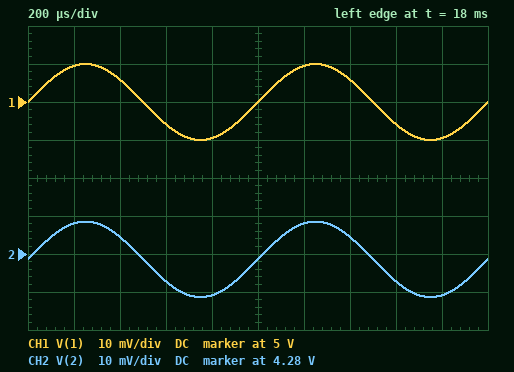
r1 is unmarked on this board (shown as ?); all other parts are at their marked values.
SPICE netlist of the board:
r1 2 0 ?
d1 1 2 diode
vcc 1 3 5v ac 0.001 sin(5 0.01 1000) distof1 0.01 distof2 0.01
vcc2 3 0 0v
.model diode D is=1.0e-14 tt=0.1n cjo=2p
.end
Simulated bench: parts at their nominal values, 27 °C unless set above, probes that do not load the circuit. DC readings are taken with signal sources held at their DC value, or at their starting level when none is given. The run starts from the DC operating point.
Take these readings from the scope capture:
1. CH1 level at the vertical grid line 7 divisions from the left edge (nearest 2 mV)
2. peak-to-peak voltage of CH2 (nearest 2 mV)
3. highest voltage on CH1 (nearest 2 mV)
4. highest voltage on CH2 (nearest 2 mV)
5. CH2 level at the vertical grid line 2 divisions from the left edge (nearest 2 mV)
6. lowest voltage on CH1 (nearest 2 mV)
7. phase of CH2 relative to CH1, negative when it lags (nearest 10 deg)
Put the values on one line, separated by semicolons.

5.006 V; 20 mV; 5.010 V; 4.288 V; 4.284 V; 4.990 V; 0 deg
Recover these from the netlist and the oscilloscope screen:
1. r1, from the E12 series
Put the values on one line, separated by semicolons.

330 Ω
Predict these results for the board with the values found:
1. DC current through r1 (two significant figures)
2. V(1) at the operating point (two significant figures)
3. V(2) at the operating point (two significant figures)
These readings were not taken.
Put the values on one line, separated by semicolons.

13 mA; 5.0 V; 4.3 V
